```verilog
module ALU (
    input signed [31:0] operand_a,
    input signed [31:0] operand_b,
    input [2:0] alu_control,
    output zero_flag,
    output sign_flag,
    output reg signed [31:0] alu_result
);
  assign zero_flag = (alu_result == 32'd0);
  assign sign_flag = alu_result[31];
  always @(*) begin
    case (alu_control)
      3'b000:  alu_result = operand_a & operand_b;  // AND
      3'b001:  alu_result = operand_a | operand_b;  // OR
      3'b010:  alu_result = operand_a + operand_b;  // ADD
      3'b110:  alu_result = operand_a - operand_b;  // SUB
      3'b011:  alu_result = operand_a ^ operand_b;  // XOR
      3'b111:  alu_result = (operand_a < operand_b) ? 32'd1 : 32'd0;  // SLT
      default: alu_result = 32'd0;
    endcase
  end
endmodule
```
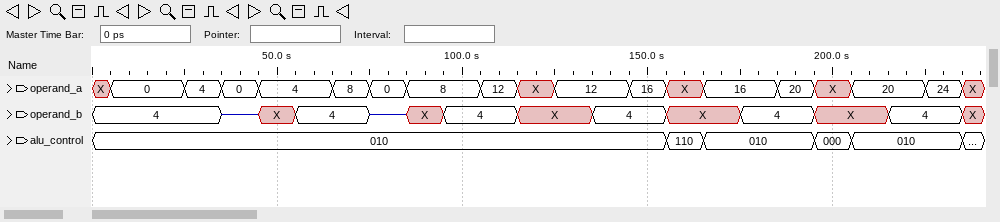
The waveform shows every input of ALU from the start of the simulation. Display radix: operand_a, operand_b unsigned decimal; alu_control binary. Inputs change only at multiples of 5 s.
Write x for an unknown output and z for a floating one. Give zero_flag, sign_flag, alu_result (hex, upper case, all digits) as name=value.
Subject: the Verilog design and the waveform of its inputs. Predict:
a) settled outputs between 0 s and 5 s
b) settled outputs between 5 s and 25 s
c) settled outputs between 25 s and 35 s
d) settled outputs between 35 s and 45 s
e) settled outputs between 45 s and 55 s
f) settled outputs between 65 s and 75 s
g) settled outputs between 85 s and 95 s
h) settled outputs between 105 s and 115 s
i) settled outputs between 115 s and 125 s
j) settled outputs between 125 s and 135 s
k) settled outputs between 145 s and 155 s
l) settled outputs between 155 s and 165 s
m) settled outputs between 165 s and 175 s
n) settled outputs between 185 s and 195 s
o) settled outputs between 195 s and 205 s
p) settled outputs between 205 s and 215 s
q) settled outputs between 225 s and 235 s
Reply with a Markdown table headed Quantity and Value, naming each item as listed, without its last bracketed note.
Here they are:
| Quantity | Value |
|---|---|
| settled outputs between 0 s and 5 s | zero_flag=x, sign_flag=x, alu_result=x |
| settled outputs between 5 s and 25 s | zero_flag=0, sign_flag=0, alu_result=00000004 |
| settled outputs between 25 s and 35 s | zero_flag=0, sign_flag=0, alu_result=00000008 |
| settled outputs between 35 s and 45 s | zero_flag=x, sign_flag=x, alu_result=x |
| settled outputs between 45 s and 55 s | zero_flag=x, sign_flag=x, alu_result=x |
| settled outputs between 65 s and 75 s | zero_flag=0, sign_flag=0, alu_result=0000000C |
| settled outputs between 85 s and 95 s | zero_flag=x, sign_flag=x, alu_result=x |
| settled outputs between 105 s and 115 s | zero_flag=0, sign_flag=0, alu_result=00000010 |
| settled outputs between 115 s and 125 s | zero_flag=x, sign_flag=x, alu_result=x |
| settled outputs between 125 s and 135 s | zero_flag=x, sign_flag=x, alu_result=x |
| settled outputs between 145 s and 155 s | zero_flag=0, sign_flag=0, alu_result=00000014 |
| settled outputs between 155 s and 165 s | zero_flag=x, sign_flag=x, alu_result=x |
| settled outputs between 165 s and 175 s | zero_flag=x, sign_flag=x, alu_result=x |
| settled outputs between 185 s and 195 s | zero_flag=0, sign_flag=0, alu_result=00000018 |
| settled outputs between 195 s and 205 s | zero_flag=x, sign_flag=x, alu_result=x |
| settled outputs between 205 s and 215 s | zero_flag=x, sign_flag=x, alu_result=x |
| settled outputs between 225 s and 235 s | zero_flag=0, sign_flag=0, alu_result=0000001C |
